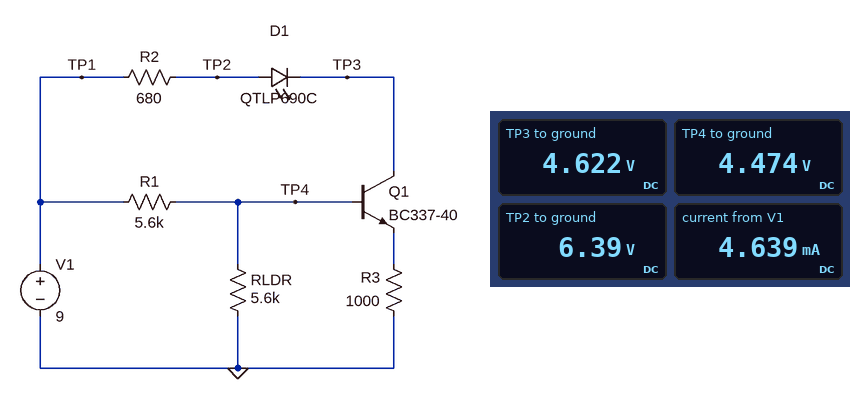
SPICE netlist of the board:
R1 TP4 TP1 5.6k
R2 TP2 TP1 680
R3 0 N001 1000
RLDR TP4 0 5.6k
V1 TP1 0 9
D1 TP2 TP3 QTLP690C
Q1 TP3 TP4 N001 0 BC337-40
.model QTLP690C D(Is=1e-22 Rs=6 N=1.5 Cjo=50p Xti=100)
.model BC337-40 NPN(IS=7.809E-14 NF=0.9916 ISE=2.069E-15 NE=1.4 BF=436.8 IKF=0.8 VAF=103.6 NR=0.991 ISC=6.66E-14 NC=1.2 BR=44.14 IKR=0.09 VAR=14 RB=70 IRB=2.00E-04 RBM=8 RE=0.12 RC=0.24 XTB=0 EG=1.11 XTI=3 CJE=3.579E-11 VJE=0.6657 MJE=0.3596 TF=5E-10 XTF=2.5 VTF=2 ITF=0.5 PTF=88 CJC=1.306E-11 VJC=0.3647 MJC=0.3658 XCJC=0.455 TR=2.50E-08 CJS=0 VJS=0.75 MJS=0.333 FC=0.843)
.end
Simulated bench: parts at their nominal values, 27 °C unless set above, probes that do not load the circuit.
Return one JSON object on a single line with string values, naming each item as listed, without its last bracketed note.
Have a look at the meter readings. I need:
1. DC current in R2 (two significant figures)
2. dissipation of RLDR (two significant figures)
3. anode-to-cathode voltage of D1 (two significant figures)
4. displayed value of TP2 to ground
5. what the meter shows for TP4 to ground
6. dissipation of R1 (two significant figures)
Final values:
{"DC current in R2": "3.8 mA", "dissipation of RLDR": "3.6 mW", "anode-to-cathode voltage of D1": "1.8 V", "displayed value of TP2 to ground": "6.39 V", "what the meter shows for TP4 to ground": "4.474 V", "dissipation of R1": "3.7 mW"}
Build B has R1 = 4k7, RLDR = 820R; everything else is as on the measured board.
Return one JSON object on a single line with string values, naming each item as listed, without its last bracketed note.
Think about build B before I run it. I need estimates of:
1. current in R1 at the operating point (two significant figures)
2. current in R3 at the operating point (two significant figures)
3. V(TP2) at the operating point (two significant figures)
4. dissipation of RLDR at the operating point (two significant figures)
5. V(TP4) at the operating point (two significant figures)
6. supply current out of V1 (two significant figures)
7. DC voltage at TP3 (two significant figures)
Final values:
{"current in R1 at the operating point": "1.6 mA", "current in R3 at the operating point": "750 µA", "V(TP2) at the operating point": "8.5 V", "dissipation of RLDR at the operating point": "2.2 mW", "V(TP4) at the operating point": "1.3 V", "supply current out of V1": "2.4 mA", "DC voltage at TP3": "6.8 V"}
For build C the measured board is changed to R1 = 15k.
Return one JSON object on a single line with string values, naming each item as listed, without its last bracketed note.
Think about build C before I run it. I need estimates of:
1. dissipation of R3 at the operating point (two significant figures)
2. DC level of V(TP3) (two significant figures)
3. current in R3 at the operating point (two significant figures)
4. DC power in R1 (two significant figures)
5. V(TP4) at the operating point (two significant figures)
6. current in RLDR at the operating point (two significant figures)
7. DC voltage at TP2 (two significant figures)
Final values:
{"dissipation of R3 at the operating point": "3.3 mW", "DC level of V(TP3)": "6.0 V", "current in R3 at the operating point": "1.8 mA", "DC power in R1": "2.9 mW", "V(TP4) at the operating point": "2.4 V", "current in RLDR at the operating point": "430 µA", "DC voltage at TP2": "7.8 V"}
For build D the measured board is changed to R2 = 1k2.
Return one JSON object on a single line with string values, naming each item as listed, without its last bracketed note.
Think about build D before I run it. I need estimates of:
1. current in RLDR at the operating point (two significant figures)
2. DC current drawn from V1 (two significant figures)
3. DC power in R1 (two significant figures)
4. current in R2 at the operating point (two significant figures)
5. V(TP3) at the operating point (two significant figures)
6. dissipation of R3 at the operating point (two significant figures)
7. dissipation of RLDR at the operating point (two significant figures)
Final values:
{"current in RLDR at the operating point": "720 µA", "DC current drawn from V1": "4.1 mA", "DC power in R1": "4.4 mW", "current in R2 at the operating point": "3.2 mA", "V(TP3) at the operating point": "3.4 V", "dissipation of R3 at the operating point": "11 mW", "dissipation of RLDR at the operating point": "2.9 mW"}
